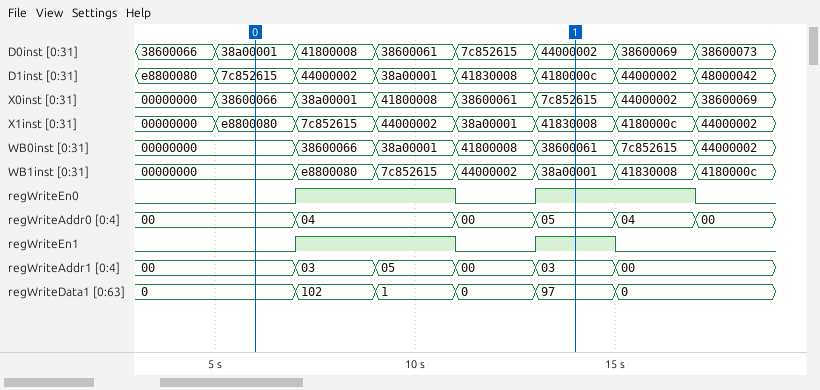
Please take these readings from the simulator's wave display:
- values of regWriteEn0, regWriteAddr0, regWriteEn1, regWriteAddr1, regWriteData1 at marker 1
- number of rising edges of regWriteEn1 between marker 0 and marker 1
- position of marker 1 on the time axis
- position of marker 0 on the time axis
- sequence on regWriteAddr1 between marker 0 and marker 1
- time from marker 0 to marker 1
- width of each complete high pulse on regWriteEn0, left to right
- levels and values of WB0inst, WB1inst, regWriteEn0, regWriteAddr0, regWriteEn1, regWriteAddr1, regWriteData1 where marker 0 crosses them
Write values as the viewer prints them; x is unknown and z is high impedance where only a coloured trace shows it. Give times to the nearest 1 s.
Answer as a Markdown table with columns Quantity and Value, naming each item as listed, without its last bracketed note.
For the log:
| Quantity | Value |
|---|---|
| values of regWriteEn0, regWriteAddr0, regWriteEn1, regWriteAddr1, regWriteData1 at marker 1 | regWriteEn0=1, regWriteAddr0=05, regWriteEn1=1, regWriteAddr1=03, regWriteData1=97 |
| number of rising edges of regWriteEn1 between marker 0 and marker 1 | 2 |
| position of marker 1 on the time axis | 14 s |
| position of marker 0 on the time axis | 6 s |
| sequence on regWriteAddr1 between marker 0 and marker 1 | 00, 03, 05, 00, 03 |
| time from marker 0 to marker 1 | 8 s |
| width of each complete high pulse on regWriteEn0, left to right | 4 s, 4 s |
| levels and values of WB0inst, WB1inst, regWriteEn0, regWriteAddr0, regWriteEn1, regWriteAddr1, regWriteData1 where marker 0 crosses them | WB0inst=00000000, WB1inst=00000000, regWriteEn0=0, regWriteAddr0=00, regWriteEn1=0, regWriteAddr1=00, regWriteData1=0 |
